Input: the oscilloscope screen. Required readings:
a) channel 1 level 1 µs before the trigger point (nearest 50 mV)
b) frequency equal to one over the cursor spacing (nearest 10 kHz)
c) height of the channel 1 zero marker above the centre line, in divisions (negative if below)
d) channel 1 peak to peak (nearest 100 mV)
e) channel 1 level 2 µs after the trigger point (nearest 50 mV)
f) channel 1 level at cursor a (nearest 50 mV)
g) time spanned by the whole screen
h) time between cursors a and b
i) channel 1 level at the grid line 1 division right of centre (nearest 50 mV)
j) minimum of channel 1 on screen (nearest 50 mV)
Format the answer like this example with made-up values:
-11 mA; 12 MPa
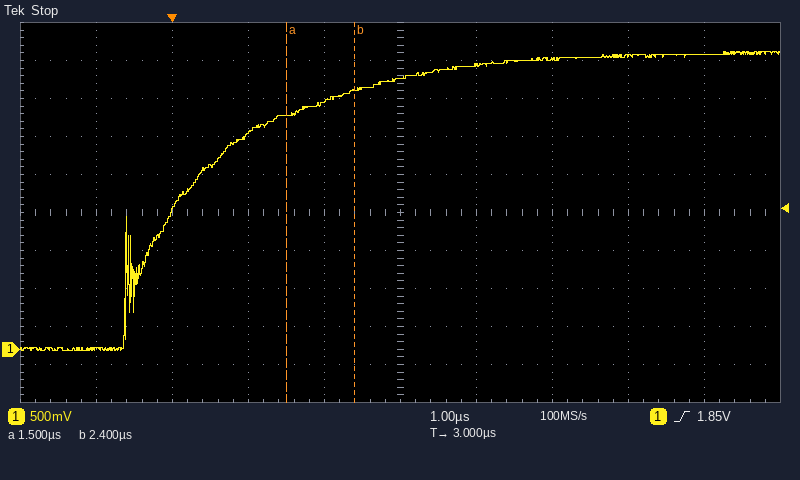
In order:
0 mV; 1.11 MHz; -3.6 div; 3.90 V; 3.25 V; 3.10 V; 10 µs; 900 ns; 3.75 V; 0 mV
